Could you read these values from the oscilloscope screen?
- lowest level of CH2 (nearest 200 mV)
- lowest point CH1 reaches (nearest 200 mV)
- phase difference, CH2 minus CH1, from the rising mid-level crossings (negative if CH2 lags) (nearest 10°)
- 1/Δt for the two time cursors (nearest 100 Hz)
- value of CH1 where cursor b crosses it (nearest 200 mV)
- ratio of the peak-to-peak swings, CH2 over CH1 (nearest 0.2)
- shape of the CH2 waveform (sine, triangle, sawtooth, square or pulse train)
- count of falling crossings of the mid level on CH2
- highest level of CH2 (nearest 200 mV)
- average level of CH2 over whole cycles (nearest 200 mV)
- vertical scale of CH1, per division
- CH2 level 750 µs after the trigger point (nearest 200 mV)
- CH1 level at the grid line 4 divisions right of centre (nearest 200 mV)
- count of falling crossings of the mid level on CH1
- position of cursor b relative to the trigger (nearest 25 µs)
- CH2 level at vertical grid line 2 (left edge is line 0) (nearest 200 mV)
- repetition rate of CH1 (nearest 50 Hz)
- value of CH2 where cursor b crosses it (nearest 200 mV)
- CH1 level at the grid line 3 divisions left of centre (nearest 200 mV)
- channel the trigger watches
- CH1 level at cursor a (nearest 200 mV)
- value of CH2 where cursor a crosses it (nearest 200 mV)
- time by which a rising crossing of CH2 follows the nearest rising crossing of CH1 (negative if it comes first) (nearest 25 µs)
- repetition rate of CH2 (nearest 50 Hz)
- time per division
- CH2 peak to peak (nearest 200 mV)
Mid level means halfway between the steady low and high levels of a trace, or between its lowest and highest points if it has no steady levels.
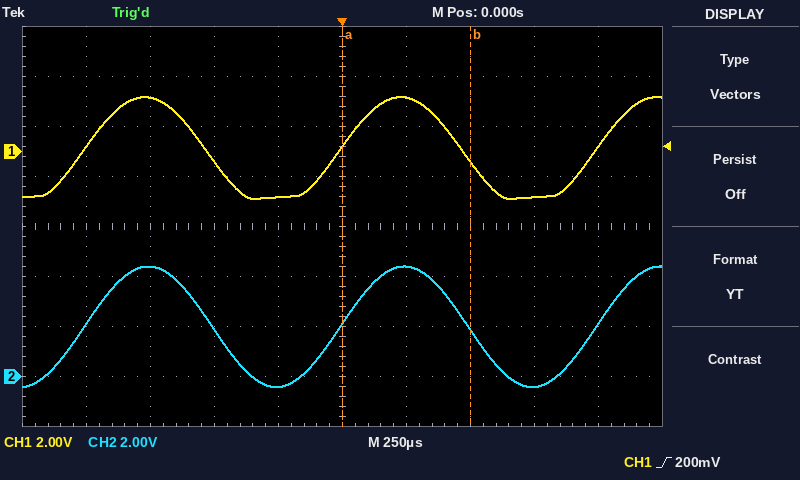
-400 mV
-1.8 V
0°
2.0 kHz
-400 mV
1.2
sine
2
4.4 V
2.0 V
2 V
-400 mV
200 mV
2
+500 µs
4.4 V
1.00 kHz
1.8 V
2.2 V
CH1
200 mV
2.2 V
0 µs
1.00 kHz
250 µs
4.8 V
